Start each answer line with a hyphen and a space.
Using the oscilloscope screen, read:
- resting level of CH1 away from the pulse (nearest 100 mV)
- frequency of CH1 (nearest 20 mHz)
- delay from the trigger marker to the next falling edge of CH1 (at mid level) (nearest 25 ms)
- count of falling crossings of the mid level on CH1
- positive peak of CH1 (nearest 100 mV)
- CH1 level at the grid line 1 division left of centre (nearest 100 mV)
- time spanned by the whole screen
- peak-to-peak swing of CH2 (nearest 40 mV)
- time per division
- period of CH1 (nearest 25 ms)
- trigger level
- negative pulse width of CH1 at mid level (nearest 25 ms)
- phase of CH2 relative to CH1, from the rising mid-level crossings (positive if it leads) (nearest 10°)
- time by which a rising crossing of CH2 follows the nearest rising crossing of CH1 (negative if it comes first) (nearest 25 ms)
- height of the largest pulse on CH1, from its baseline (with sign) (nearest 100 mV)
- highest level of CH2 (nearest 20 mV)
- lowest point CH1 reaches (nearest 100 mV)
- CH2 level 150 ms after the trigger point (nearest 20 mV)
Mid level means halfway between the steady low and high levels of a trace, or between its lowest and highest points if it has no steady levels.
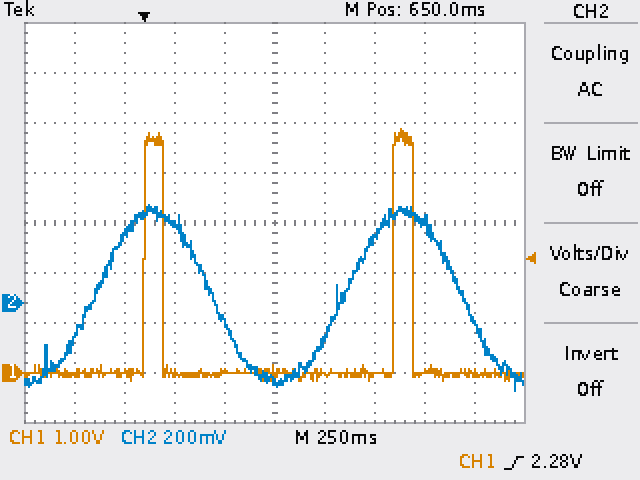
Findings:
- 0.0 V
- 800 mHz
- 100 ms
- 2
- 4.9 V
- 0.0 V
- 2.5 s
- 760 mV
- 250 ms
- 1.250 s
- 2.28 V
- 1.150 s
- +70°
- -250 ms
- +4.9 V
- 400 mV
- -200 mV
- 320 mV
